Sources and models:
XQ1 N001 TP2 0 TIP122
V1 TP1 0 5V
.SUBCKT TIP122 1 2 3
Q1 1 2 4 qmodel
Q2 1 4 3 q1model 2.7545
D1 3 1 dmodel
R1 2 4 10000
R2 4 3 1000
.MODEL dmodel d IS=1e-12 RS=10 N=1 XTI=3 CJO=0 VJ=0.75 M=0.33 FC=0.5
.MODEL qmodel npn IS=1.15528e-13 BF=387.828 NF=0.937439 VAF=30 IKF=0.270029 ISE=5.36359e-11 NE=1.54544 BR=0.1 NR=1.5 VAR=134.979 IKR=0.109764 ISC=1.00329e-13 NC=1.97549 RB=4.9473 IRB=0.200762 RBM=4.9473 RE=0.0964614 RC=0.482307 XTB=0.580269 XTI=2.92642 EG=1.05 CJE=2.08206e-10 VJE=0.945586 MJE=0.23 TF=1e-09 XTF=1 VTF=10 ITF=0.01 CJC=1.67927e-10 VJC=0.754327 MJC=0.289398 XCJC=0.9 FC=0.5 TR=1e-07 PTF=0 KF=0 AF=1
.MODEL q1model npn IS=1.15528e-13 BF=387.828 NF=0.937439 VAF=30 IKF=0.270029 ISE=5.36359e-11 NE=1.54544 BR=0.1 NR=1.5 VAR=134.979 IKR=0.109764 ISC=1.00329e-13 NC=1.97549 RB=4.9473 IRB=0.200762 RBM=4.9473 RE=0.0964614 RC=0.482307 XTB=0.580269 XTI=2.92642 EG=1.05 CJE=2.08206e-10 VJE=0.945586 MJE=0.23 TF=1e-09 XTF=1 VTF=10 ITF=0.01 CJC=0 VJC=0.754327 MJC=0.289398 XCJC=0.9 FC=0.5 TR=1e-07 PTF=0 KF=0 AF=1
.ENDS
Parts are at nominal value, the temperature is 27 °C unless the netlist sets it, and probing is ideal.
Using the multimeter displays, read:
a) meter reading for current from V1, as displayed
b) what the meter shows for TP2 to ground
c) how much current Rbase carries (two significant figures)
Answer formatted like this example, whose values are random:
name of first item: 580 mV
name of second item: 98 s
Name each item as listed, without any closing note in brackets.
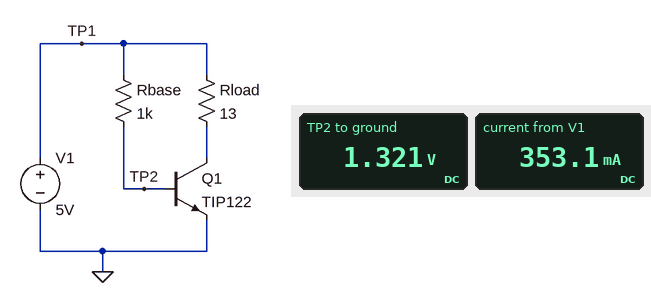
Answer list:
meter reading for current from V1, as displayed: 353.1 mA
what the meter shows for TP2 to ground: 1.321 V
how much current Rbase carries: 3.7 mA
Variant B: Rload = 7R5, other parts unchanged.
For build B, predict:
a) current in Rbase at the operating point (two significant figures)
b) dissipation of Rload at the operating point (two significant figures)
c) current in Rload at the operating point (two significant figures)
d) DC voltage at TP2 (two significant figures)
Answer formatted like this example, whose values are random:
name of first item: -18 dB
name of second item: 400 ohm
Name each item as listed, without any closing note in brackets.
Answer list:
current in Rbase at the operating point: 3.6 mA
dissipation of Rload at the operating point: 2.7 W
current in Rload at the operating point: 600 mA
DC voltage at TP2: 1.4 V
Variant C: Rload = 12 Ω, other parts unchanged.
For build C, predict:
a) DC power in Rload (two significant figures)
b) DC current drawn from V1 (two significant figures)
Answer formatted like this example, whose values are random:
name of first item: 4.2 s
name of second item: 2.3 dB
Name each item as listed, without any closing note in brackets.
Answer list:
DC power in Rload: 1.7 W
DC current drawn from V1: 380 mA
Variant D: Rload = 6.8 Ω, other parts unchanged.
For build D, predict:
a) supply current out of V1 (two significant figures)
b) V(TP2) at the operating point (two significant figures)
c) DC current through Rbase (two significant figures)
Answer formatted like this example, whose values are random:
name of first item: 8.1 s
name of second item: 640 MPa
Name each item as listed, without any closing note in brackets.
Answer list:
supply current out of V1: 660 mA
V(TP2) at the operating point: 1.4 V
DC current through Rbase: 3.6 mA
